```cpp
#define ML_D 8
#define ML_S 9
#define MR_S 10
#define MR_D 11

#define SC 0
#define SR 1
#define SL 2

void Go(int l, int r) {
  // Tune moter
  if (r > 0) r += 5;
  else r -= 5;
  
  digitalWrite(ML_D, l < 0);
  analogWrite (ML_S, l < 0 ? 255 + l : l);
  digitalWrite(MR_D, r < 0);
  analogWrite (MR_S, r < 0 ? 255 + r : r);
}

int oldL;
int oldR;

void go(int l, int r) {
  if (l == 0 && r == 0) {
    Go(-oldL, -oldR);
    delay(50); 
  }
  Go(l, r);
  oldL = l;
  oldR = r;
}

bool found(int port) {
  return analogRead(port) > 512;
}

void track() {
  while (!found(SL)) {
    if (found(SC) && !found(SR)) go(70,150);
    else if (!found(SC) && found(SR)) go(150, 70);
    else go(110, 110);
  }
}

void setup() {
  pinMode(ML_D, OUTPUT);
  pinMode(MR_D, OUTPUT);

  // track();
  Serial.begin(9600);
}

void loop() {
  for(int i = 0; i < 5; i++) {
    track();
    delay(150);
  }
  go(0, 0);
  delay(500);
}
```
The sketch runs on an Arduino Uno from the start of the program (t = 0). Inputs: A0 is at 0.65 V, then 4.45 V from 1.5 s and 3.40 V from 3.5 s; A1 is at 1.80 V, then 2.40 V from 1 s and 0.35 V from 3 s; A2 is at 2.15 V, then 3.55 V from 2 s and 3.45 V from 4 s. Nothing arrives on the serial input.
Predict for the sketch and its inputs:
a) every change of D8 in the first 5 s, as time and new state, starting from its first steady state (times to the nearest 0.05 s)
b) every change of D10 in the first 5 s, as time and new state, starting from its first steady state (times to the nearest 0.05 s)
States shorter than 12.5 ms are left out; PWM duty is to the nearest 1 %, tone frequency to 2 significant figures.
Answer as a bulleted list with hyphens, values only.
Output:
- 0 s low; 2.75 s high; 2.8 s low
- 0 s PWM 45 %; 1.5 s PWM 61 %; 2.75 s PWM 39 %; 2.8 s PWM 98 %
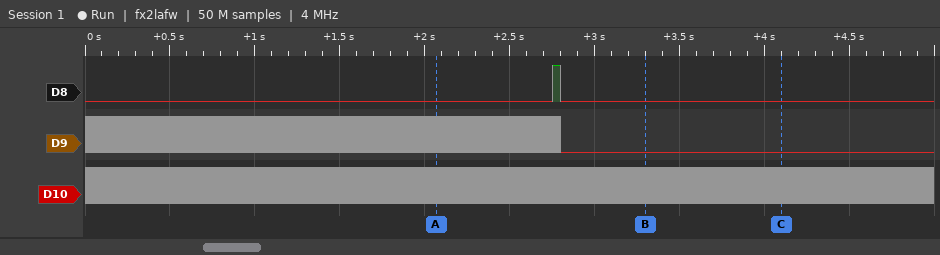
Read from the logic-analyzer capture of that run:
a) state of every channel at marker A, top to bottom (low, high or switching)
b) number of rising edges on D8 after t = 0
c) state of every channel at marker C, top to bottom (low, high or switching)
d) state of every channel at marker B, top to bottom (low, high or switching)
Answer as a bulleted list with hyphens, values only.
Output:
- D8 low, D9 switching, D10 switching
- 1
- D8 low, D9 low, D10 switching
- D8 low, D9 low, D10 switching
